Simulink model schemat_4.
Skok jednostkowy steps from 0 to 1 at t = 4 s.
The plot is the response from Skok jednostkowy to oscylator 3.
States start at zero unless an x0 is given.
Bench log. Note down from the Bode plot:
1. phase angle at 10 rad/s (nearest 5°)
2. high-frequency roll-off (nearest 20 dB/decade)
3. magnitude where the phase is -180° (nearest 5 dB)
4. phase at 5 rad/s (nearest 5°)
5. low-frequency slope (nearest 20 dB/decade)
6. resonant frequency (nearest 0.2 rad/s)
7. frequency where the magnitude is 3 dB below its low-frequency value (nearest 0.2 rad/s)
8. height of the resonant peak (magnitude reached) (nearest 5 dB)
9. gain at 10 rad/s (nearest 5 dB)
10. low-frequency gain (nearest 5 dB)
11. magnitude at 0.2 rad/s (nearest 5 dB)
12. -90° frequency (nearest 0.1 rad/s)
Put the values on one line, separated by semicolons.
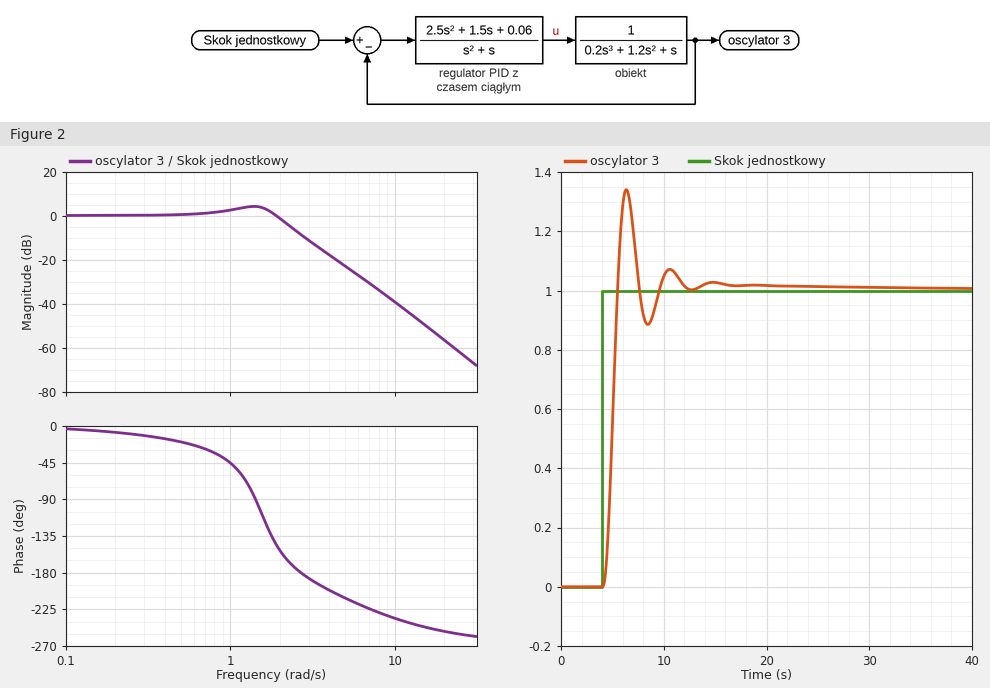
-235°; -60 dB/decade; -10 dB; -210°; 0 dB/decade; 1.4 rad/s; 2.2 rad/s; 5 dB; -40 dB; 0 dB; 0 dB; 1.4 rad/s
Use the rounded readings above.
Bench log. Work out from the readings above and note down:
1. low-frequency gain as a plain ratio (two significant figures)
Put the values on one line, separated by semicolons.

1.0
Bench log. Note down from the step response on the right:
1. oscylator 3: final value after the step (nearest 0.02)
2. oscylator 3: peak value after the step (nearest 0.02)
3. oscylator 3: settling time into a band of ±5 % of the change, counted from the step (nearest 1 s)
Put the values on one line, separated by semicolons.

1.00; 1.34; 7 s
